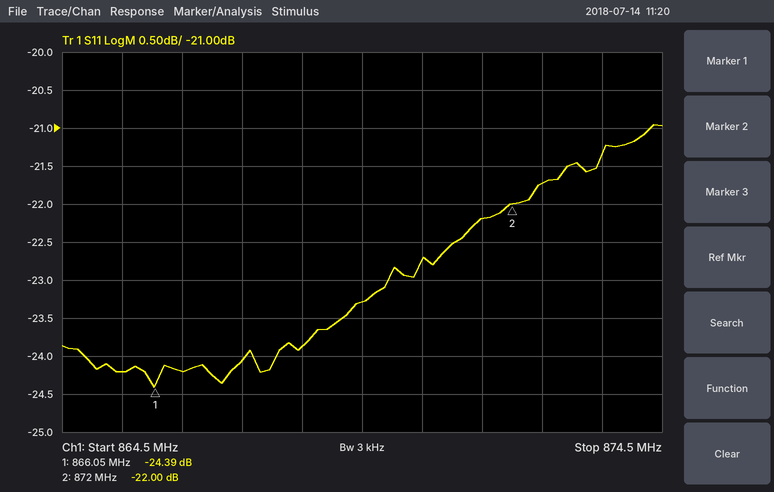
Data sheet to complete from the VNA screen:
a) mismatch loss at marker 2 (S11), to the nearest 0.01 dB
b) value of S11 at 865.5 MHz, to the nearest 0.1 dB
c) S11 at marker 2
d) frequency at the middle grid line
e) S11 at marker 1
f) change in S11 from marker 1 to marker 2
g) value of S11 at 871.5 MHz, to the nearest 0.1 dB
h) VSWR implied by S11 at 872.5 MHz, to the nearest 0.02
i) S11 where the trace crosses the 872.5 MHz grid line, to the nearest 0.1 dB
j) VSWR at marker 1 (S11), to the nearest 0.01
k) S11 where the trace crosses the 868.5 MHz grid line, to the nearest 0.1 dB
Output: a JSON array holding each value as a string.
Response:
["0.03 dB", "-24.2 dB", "-22.00 dB", "869.5 MHz", "-24.39 dB", "2.39 dB", "-22.2 dB", "1.18", "-21.7 dB", "1.13", "-23.9 dB"]
